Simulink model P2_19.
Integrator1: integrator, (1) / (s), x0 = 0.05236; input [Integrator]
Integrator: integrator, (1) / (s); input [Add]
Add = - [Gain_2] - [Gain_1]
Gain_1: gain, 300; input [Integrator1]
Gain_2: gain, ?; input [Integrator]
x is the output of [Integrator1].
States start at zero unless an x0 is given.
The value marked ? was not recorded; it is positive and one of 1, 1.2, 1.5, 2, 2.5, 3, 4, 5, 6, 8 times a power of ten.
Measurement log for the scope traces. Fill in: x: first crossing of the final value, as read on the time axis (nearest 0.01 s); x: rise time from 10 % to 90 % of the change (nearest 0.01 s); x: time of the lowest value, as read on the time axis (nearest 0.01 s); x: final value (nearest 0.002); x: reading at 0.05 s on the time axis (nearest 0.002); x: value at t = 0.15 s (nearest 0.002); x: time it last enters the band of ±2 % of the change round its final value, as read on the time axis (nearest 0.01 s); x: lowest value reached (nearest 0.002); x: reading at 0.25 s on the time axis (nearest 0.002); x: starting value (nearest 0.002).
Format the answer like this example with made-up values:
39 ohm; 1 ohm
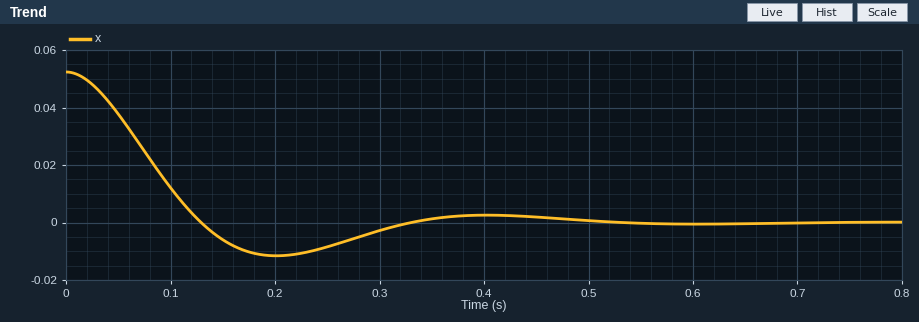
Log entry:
0.13 s; 0.09 s; 0.20 s; 0.000; 0.038; -0.006; 0.48 s; -0.012; -0.008; 0.052
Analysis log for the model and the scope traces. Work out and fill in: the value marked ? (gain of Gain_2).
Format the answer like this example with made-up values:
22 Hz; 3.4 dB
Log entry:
15
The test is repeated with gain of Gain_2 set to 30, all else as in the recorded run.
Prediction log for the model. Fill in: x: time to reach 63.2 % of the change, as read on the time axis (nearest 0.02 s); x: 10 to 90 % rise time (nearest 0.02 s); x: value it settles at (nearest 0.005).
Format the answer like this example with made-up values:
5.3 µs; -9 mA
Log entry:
0.12 s; 0.16 s; 0.000
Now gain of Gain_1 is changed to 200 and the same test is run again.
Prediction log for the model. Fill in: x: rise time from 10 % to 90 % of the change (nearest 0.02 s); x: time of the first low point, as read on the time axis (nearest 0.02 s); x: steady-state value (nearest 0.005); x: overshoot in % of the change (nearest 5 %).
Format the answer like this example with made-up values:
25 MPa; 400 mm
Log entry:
0.12 s; 0.26 s; 0.000; 15 %
